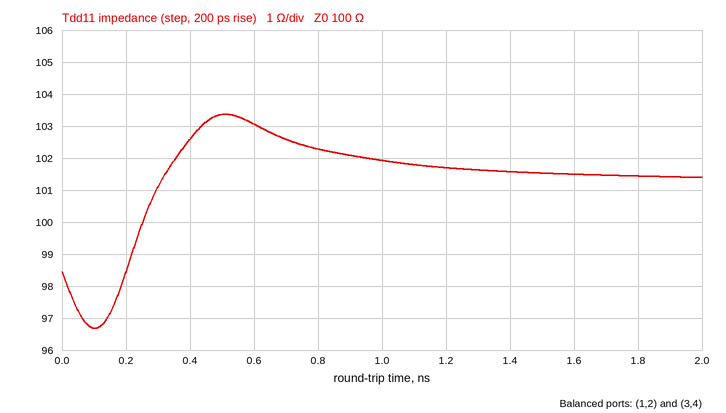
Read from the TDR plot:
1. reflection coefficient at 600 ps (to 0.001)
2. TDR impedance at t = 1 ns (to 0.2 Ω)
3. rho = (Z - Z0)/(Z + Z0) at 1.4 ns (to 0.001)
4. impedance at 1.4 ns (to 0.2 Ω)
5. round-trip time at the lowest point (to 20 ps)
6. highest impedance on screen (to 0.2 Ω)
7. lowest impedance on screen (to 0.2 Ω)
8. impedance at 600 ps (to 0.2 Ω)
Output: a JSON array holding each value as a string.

["+0.015", "102.0 Ω", "+0.008", "101.6 Ω", "100 ps", "103.4 Ω", "96.6 Ω", "103.0 Ω"]
